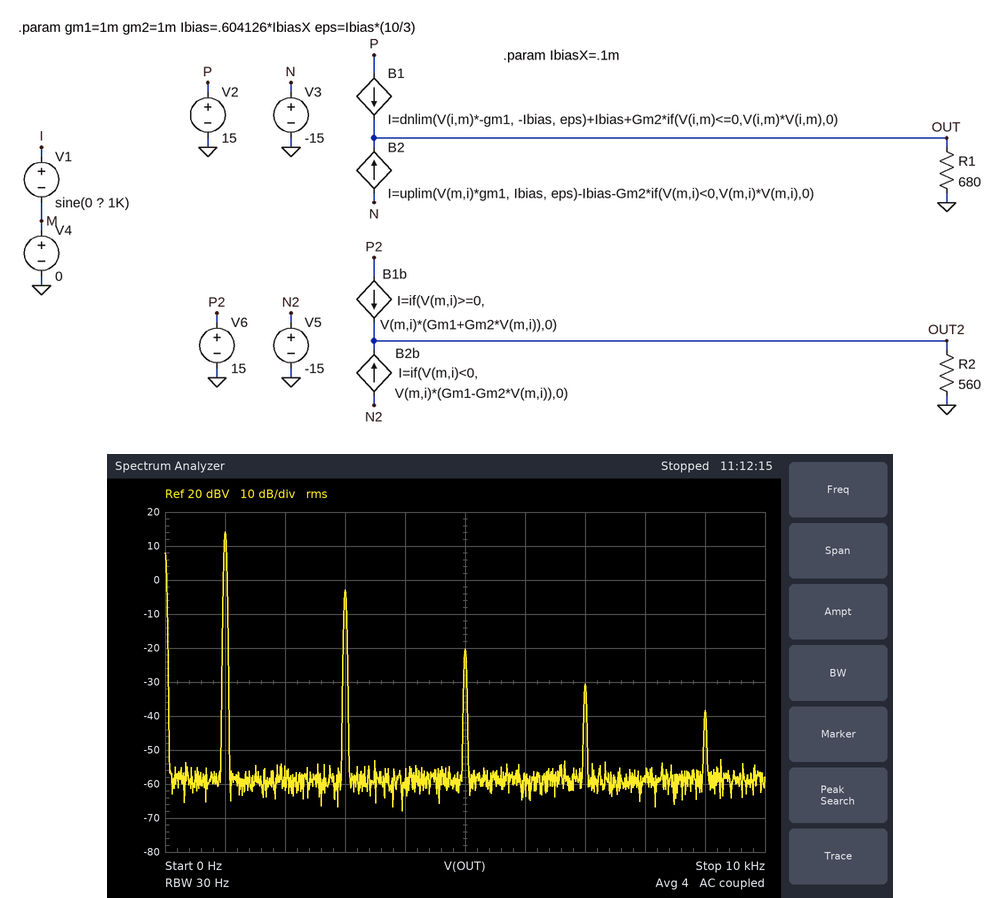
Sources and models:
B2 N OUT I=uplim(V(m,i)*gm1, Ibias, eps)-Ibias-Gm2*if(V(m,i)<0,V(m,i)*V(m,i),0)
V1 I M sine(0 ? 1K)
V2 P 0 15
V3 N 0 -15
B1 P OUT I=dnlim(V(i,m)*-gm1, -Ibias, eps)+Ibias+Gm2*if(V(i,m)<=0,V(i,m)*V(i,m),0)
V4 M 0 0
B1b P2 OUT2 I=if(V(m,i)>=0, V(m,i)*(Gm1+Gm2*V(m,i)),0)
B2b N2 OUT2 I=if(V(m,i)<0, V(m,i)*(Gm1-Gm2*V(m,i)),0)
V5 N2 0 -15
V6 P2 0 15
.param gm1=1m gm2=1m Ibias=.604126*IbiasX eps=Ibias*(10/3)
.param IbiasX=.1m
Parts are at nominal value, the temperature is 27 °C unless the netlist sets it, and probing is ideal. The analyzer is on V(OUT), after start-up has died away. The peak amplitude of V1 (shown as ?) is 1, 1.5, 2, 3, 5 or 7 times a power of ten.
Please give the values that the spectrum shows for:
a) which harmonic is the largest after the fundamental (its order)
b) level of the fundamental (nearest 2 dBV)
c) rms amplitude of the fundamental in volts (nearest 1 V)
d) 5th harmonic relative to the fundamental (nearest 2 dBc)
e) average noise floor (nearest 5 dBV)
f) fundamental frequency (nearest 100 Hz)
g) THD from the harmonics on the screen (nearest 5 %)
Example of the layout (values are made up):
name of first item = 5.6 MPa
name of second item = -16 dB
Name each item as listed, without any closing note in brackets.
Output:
which harmonic is the largest after the fundamental = 3
level of the fundamental = 14 dBV
rms amplitude of the fundamental in volts = 5 V
5th harmonic relative to the fundamental = -34 dBc
average noise floor = -60 dBV
fundamental frequency = 1.0 kHz
THD from the harmonics on the screen = 15 %
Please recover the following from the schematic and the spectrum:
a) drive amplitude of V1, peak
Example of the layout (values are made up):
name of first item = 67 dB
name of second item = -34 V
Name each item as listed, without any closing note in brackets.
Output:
drive amplitude of V1, peak = 3 V
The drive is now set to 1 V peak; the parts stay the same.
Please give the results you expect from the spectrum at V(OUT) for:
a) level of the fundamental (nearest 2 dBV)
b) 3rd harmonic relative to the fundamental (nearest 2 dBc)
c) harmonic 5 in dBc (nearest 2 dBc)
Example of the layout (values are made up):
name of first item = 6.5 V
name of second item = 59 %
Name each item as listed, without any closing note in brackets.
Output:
level of the fundamental = 0 dBV
3rd harmonic relative to the fundamental = -22 dBc
harmonic 5 in dBc = -44 dBc
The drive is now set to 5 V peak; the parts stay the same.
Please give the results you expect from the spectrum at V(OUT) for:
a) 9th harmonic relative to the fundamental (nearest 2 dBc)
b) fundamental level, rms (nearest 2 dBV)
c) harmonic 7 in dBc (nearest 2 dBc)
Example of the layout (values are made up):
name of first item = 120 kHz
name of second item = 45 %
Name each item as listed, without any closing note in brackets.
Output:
9th harmonic relative to the fundamental = -50 dBc
fundamental level, rms = 22 dBV
harmonic 7 in dBc = -42 dBc
